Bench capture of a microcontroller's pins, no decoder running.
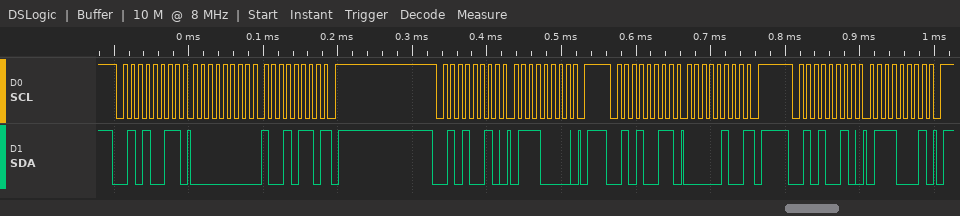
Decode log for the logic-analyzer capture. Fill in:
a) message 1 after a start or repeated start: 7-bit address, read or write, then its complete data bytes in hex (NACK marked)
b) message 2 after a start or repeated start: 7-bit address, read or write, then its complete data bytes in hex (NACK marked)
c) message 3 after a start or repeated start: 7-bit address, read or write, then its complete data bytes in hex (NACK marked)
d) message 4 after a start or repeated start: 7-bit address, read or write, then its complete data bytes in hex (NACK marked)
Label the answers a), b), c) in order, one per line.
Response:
a) 0x29 read: 00 96 NACK
b) 0x29 write: 70
c) 0x29 read: 04 NACK
d) 0x29 write: 71
